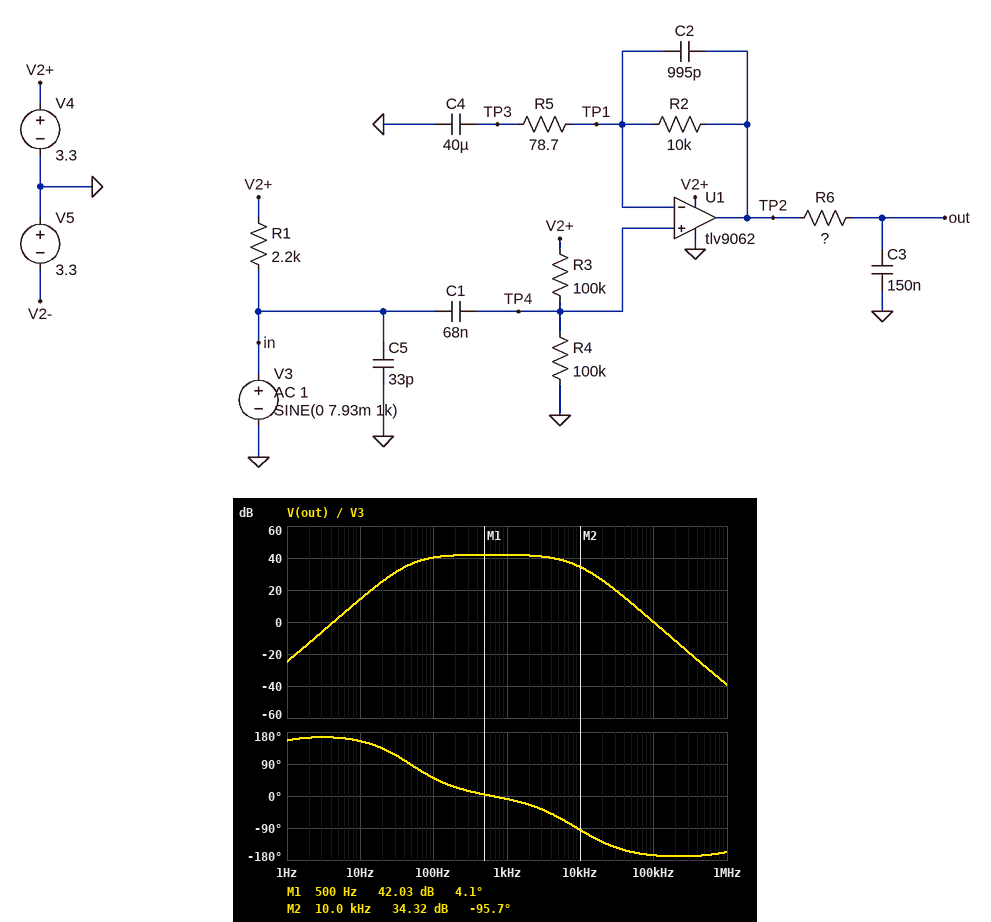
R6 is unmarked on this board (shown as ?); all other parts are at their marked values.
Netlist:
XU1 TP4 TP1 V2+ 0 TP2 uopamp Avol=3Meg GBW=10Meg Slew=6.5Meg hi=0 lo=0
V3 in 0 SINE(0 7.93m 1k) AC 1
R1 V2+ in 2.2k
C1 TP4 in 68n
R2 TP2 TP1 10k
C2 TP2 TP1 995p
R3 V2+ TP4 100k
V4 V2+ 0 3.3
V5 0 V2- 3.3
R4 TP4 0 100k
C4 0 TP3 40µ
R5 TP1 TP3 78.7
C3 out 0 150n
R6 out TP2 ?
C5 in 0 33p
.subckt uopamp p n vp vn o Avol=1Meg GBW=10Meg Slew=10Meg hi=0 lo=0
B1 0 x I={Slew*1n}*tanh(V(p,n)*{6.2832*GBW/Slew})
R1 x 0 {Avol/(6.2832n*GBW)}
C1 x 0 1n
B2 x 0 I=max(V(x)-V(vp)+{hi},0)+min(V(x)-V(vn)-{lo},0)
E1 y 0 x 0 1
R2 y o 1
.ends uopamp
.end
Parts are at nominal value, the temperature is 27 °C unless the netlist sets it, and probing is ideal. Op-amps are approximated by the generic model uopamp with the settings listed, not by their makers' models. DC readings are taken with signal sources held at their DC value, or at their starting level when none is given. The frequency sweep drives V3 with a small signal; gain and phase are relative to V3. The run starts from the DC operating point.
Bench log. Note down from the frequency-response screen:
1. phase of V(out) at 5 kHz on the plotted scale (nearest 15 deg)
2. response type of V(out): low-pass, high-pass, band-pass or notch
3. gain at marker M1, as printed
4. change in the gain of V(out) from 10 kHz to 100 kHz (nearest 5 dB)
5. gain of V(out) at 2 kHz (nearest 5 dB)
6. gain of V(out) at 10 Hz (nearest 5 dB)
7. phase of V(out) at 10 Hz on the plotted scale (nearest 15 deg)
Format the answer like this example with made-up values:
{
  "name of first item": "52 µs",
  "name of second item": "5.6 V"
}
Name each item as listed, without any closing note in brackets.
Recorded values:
{
  "phase of V(out) at 5 kHz on the plotted scale": "-60 deg",
  "response type of V(out): low-pass, high-pass, band-pass or notch": "band-pass",
  "gain at marker M1, as printed": "42.03 dB",
  "change in the gain of V(out) from 10 kHz to 100 kHz": "-35 dB",
  "gain of V(out) at 2 kHz": "40 dB",
  "gain of V(out) at 10 Hz": "15 dB",
  "phase of V(out) at 10 Hz on the plotted scale": "150 deg"
}
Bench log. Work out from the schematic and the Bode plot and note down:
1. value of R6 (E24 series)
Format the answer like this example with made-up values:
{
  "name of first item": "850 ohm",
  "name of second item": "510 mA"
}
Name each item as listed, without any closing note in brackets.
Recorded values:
{
  "value of R6": "180 Ω"
}
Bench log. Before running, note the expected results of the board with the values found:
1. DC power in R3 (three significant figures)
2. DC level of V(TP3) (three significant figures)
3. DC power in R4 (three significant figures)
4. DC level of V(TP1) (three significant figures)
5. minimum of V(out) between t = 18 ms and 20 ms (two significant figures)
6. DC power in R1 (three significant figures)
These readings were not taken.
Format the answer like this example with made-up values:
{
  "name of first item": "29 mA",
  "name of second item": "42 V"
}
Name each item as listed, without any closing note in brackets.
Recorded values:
{
  "DC power in R3": "27.2 µW",
  "DC level of V(TP3)": "1.65 V",
  "DC power in R4": "27.2 µW",
  "DC level of V(TP1)": "1.65 V",
  "minimum of V(out) between t = 18 ms and 20 ms": "650 mV",
  "DC power in R1": "4.95 mW"
}
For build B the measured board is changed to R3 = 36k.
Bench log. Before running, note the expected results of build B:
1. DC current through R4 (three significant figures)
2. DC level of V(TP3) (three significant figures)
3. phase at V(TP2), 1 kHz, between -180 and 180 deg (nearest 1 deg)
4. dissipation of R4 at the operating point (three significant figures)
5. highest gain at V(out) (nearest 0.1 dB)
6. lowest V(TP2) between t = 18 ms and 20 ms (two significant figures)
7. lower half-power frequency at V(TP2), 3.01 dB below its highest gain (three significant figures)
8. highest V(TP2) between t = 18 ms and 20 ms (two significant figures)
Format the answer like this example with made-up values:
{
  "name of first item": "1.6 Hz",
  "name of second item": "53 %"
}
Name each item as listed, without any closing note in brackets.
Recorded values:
{
  "DC current through R4": "24.3 µA",
  "DC level of V(TP3)": "2.43 V",
  "phase at V(TP2), 1 kHz, between -180 and 180 deg": "4 deg",
  "dissipation of R4 at the operating point": "58.9 µW",
  "highest gain at V(out)": "42.0 dB",
  "lowest V(TP2) between t = 18 ms and 20 ms": "1.4 V",
  "lower half-power frequency at V(TP2), 3.01 dB below its highest gain": "108 Hz",
  "highest V(TP2) between t = 18 ms and 20 ms": "3.3 V"
}
